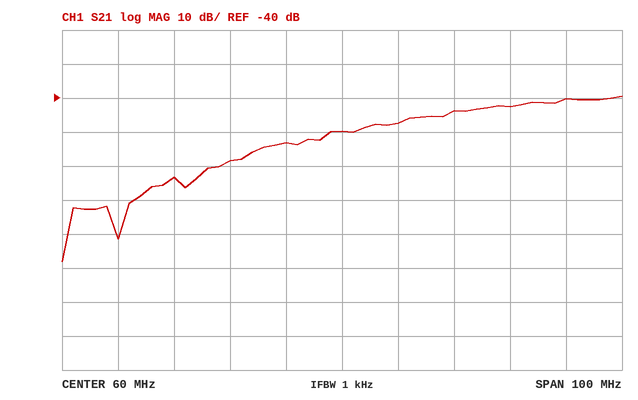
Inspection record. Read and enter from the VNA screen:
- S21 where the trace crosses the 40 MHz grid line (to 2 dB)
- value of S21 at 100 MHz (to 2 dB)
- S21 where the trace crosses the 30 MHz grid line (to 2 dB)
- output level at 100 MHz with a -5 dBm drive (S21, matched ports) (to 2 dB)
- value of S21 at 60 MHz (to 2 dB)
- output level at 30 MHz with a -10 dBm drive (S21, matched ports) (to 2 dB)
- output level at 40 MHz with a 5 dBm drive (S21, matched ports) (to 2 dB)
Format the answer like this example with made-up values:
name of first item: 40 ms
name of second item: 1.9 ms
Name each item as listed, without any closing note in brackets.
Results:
S21 where the trace crosses the 40 MHz grid line: -58 dB
value of S21 at 100 MHz: -40 dB
S21 where the trace crosses the 30 MHz grid line: -64 dB
output level at 100 MHz with a -5 dBm drive (S21, matched ports): -46 dBm
value of S21 at 60 MHz: -50 dB
output level at 30 MHz with a -10 dBm drive (S21, matched ports): -74 dBm
output level at 40 MHz with a 5 dBm drive (S21, matched ports): -54 dBm
